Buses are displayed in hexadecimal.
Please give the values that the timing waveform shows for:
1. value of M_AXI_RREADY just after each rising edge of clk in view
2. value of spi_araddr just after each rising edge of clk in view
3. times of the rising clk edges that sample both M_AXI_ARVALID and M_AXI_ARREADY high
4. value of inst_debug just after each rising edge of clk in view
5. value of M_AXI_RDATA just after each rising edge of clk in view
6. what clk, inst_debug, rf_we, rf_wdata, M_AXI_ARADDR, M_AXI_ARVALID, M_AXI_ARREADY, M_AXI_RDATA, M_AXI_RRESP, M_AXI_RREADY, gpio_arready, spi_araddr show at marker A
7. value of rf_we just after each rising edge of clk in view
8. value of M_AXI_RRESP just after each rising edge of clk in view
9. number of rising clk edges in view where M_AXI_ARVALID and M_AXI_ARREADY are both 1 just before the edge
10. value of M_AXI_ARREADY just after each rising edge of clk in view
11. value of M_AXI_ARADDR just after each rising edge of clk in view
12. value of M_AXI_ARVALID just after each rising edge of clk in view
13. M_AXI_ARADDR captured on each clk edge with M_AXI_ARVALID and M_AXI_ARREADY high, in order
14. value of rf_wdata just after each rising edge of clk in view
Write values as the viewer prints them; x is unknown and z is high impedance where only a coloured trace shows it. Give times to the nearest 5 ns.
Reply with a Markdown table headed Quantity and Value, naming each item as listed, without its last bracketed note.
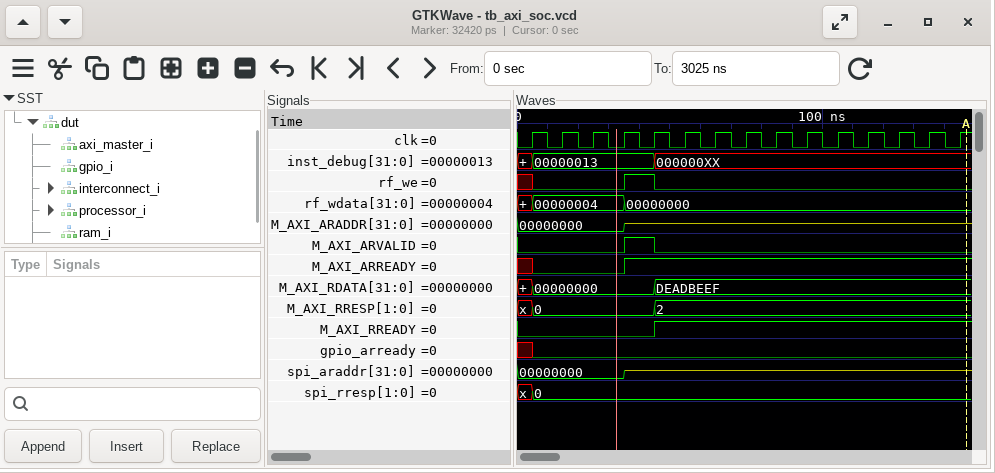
| Quantity | Value |
|---|---|
| value of M_AXI_RREADY just after each rising edge of clk in view | 0 0 0 0 1 1 1 1 1 1 1 1 1 1 1 |
| value of spi_araddr just after each rising edge of clk in view | 00000000, 00000000, 00000000, z, z, z, z, z, z, z, z, z, z, z, z |
| times of the rising clk edges that sample both M_AXI_ARVALID and M_AXI_ARREADY high | 45 ns |
| value of inst_debug just after each rising edge of clk in view | 00000013, 00000013, 00000013, 00000013, 000000XX, 000000XX, 000000XX, 000000XX, 000000XX, 000000XX, 000000XX, 000000XX, 000000XX, 000000XX, 000000XX |
| value of M_AXI_RDATA just after each rising edge of clk in view | 00000000, 00000000, 00000000, 00000000, DEADBEEF, DEADBEEF, DEADBEEF, DEADBEEF, DEADBEEF, DEADBEEF, DEADBEEF, DEADBEEF, DEADBEEF, DEADBEEF, DEADBEEF |
| what clk, inst_debug, rf_we, rf_wdata, M_AXI_ARADDR, M_AXI_ARVALID, M_AXI_ARREADY, M_AXI_RDATA, M_AXI_RRESP, M_AXI_RREADY, gpio_arready, spi_araddr show at marker A | clk=1, inst_debug=000000XX, rf_we=0, rf_wdata=00000000, M_AXI_ARADDR=z, M_AXI_ARVALID=0, M_AXI_ARREADY=1, M_AXI_RDATA=DEADBEEF, M_AXI_RRESP=2, M_AXI_RREADY=1, gpio_arready=0, spi_araddr=z |
| value of rf_we just after each rising edge of clk in view | 0 0 0 1 0 0 0 0 0 0 0 0 0 0 0 |
| value of M_AXI_RRESP just after each rising edge of clk in view | 0, 0, 0, 0, 2, 2, 2, 2, 2, 2, 2, 2, 2, 2, 2 |
| number of rising clk edges in view where M_AXI_ARVALID and M_AXI_ARREADY are both 1 just before the edge | 1 |
| value of M_AXI_ARREADY just after each rising edge of clk in view | 0 0 0 1 1 1 1 1 1 1 1 1 1 1 1 |
| value of M_AXI_ARADDR just after each rising edge of clk in view | 00000000, 00000000, 00000000, z, z, z, z, z, z, z, z, z, z, z, z |
| value of M_AXI_ARVALID just after each rising edge of clk in view | 0 0 0 1 0 0 0 0 0 0 0 0 0 0 0 |
| M_AXI_ARADDR captured on each clk edge with M_AXI_ARVALID and M_AXI_ARREADY high, in order | z |
| value of rf_wdata just after each rising edge of clk in view | 00000004, 00000004, 00000004, 00000000, 00000000, 00000000, 00000000, 00000000, 00000000, 00000000, 00000000, 00000000, 00000000, 00000000, 00000000 |
